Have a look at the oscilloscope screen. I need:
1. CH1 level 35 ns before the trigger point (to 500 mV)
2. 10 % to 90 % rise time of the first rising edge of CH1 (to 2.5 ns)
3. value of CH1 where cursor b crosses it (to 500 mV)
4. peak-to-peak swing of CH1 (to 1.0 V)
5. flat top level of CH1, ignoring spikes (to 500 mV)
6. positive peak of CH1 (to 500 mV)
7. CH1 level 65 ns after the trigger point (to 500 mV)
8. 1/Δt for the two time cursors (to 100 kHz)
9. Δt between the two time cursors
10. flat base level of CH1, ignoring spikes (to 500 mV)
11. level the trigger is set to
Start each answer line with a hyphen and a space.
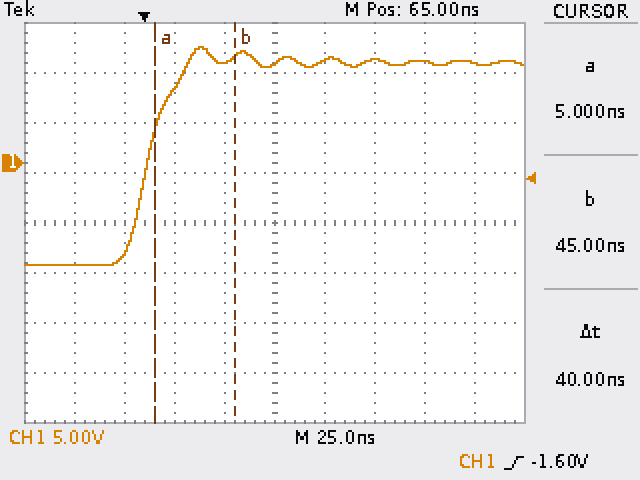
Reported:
- -10.0 V
- 25.0 ns
- 10.5 V
- 22.0 V
- 10.0 V
- 11.5 V
- 10.0 V
- 25.0 MHz
- 40 ns
- -10.0 V
- -1.60 V
